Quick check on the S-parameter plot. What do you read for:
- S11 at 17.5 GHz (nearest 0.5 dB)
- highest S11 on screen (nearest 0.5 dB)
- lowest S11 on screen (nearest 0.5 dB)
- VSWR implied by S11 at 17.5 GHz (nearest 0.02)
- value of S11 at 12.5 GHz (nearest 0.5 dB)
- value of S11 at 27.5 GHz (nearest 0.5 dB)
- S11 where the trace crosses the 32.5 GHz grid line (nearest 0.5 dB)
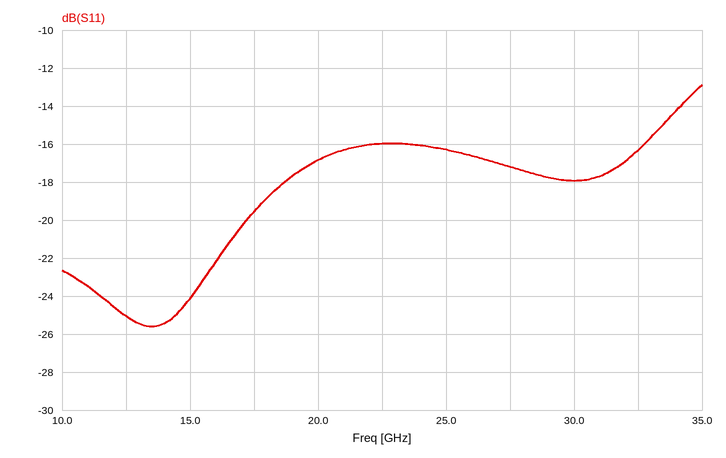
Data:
-19.5 dB
-13.0 dB
-25.5 dB
1.24
-25.0 dB
-17.0 dB
-16.5 dB
